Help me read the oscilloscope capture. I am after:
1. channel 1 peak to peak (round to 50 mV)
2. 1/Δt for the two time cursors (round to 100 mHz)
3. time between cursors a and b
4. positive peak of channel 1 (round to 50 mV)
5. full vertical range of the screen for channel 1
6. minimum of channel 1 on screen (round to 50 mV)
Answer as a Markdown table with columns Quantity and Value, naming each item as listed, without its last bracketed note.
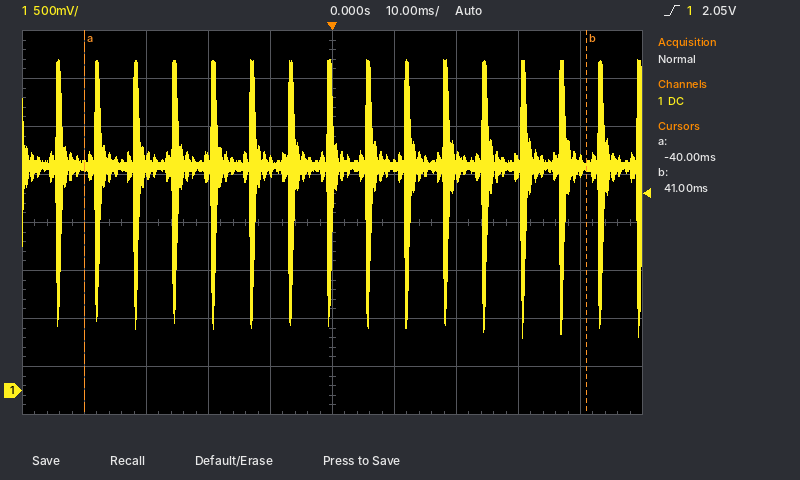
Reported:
| Quantity | Value |
|---|---|
| channel 1 peak to peak | 2.90 V |
| 1/Δt for the two time cursors | 12.3 Hz |
| time between cursors a and b | 81 ms |
| positive peak of channel 1 | 3.45 V |
| full vertical range of the screen for channel 1 | 4 V |
| minimum of channel 1 on screen | 550 mV |
